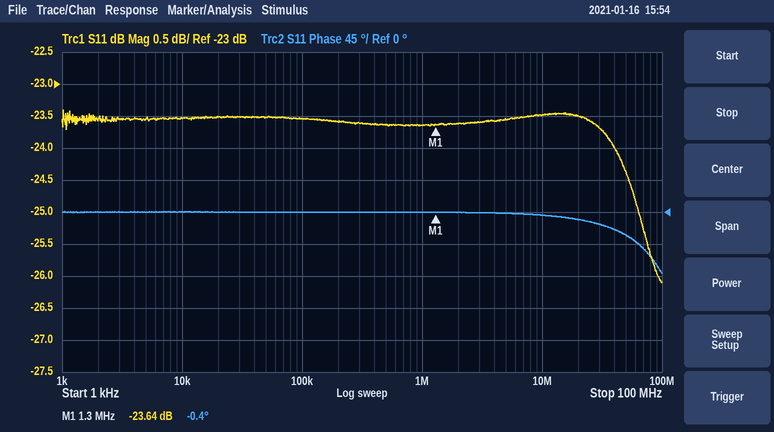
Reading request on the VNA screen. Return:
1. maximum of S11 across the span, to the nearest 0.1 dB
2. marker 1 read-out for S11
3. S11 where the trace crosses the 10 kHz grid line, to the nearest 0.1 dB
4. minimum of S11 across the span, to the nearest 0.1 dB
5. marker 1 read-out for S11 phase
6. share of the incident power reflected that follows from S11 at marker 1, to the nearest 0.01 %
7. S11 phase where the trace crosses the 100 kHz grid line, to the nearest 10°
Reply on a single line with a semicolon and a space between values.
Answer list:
-23.4 dB; -23.64 dB; -23.5 dB; -26.1 dB; -0.4°; 0.43 %; 0°
